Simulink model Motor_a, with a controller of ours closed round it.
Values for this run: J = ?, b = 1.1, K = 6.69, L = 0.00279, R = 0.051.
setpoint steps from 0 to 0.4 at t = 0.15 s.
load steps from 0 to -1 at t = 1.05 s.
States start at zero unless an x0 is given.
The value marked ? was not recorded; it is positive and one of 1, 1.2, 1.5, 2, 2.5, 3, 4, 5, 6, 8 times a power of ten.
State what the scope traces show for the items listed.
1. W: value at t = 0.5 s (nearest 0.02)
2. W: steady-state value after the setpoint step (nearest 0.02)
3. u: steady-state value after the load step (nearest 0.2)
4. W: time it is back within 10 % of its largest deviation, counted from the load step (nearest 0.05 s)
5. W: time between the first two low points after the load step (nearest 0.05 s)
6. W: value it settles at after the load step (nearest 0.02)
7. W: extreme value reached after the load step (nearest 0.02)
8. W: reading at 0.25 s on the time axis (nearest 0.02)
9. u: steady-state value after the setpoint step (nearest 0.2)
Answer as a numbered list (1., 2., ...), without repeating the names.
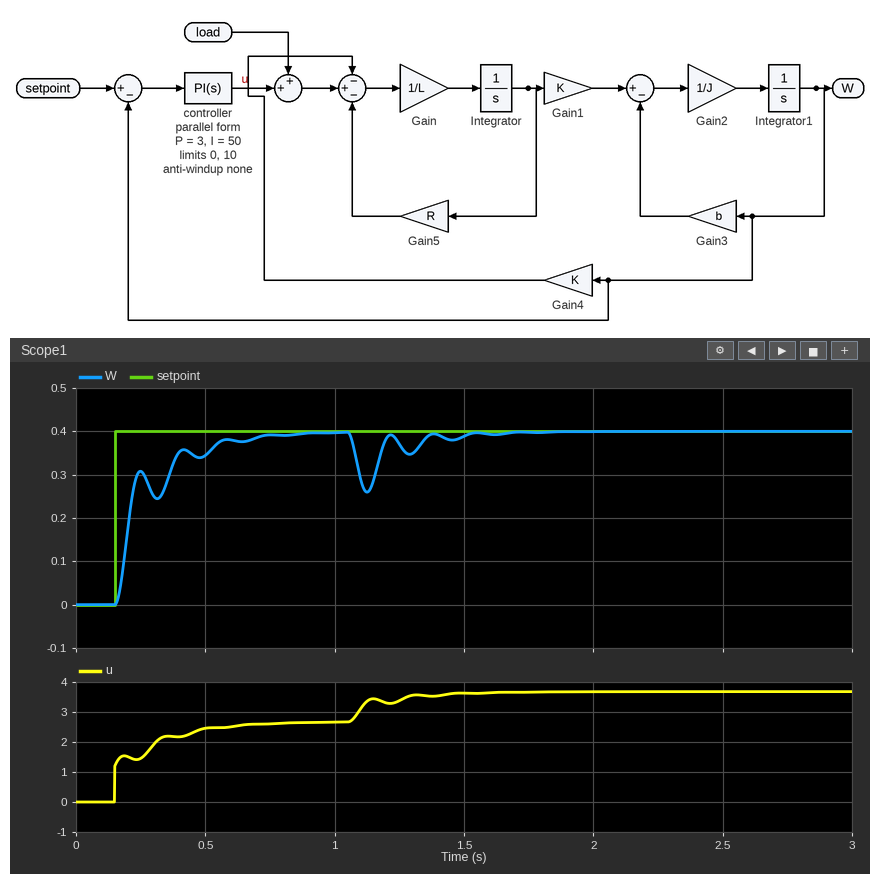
1. 0.34
2. 0.40
3. 3.6
4. 0.45 s
5. 0.15 s
6. 0.40
7. 0.26
8. 0.30
9. 2.6
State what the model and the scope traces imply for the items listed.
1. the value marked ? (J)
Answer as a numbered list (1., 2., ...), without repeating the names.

1. 15
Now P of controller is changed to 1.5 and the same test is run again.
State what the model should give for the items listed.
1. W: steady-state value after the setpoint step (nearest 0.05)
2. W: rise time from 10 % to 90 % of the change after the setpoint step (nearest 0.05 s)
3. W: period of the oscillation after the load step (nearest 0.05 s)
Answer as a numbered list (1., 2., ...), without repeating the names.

1. 0.40
2. 0.25 s
3. 0.20 s
